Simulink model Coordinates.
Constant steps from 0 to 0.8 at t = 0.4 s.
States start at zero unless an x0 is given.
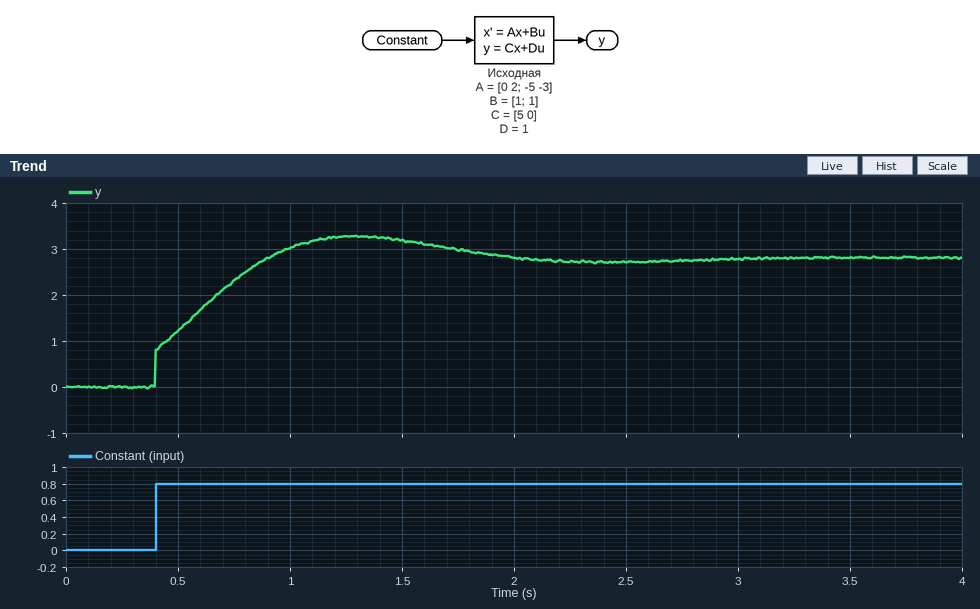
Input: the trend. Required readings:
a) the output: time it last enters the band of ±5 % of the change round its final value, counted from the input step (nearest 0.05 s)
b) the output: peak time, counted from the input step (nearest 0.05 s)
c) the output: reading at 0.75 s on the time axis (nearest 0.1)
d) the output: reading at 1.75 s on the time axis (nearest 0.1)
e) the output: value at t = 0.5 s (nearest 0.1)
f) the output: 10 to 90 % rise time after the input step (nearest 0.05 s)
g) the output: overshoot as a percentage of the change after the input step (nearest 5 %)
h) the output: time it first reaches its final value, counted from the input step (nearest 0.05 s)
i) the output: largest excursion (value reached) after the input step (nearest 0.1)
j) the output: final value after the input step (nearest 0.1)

1.40 s
0.90 s
2.3
3.0
1.2
0.40 s
15 %
0.50 s
3.3
2.8
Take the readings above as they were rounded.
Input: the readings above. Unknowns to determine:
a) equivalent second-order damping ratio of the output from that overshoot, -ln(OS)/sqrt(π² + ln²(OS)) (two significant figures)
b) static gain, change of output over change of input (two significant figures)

0.52
3.5
